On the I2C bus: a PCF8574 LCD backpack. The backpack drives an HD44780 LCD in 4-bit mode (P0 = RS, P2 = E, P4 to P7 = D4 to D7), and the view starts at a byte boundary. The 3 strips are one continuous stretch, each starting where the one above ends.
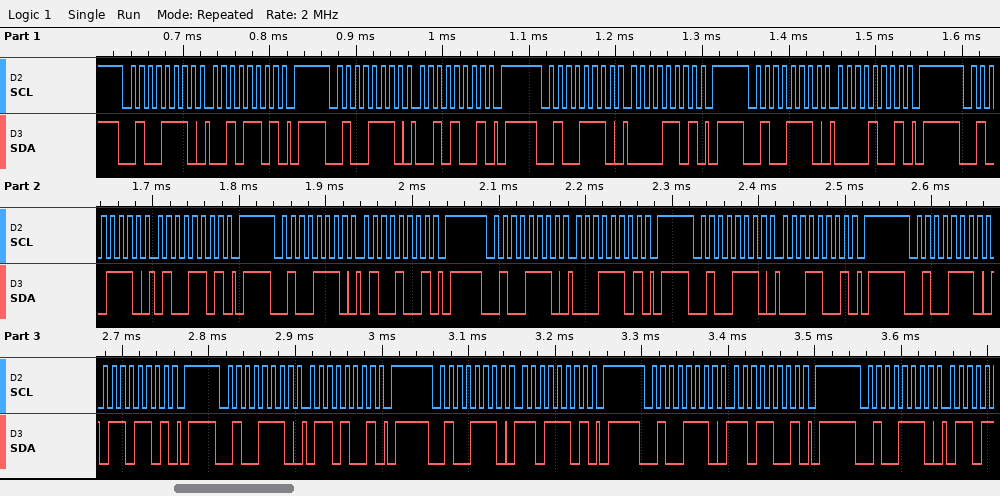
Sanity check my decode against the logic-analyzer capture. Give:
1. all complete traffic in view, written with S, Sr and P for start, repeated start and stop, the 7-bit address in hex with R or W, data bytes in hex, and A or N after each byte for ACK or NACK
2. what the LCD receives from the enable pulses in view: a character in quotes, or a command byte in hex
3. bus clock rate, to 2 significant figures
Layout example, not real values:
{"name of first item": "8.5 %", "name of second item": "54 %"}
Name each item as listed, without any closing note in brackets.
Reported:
{"all complete traffic in view, written with S, Sr and P for start, repeated start and stop, the 7-bit address in hex with R or W, data bytes in hex, and A or N after each byte for ACK or NACK": "S 27W A 2D A P S 27W A 29 A P S 27W A 0D A P S 27W A 09 A P S 27W A 4D A P S 27W A 49 A P S 27W A 1D A P S 27W A 19 A P S 27W A 6D A P S 27W A 69 A P S 27W A DD A P S 27W A D9 A P S 27W A", "what the LCD receives from the enable pulses in view: a character in quotes, or a command byte in hex": "' ' 'A' 'm'", "bus clock rate, to 2 significant figures": "100 kHz"}
